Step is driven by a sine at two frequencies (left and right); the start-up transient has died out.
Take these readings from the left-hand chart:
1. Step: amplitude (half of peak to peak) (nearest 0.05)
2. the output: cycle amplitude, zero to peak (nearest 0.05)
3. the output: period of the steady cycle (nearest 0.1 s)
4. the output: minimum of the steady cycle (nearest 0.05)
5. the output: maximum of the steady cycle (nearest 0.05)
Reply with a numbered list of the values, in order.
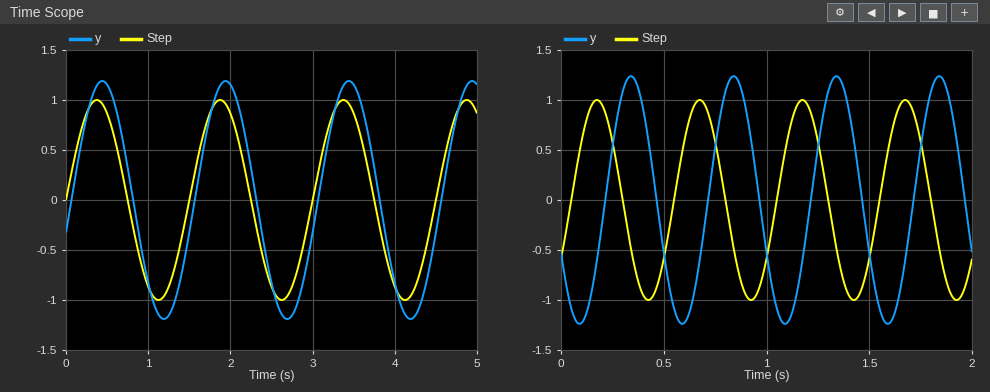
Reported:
1. 1.00
2. 1.20
3. 1.5 s
4. -1.20
5. 1.20
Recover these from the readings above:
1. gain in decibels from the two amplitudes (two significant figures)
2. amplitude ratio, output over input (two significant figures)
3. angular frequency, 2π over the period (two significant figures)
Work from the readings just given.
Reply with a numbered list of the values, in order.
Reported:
1. 1.6 dB
2. 1.2
3. 4.2 rad/s
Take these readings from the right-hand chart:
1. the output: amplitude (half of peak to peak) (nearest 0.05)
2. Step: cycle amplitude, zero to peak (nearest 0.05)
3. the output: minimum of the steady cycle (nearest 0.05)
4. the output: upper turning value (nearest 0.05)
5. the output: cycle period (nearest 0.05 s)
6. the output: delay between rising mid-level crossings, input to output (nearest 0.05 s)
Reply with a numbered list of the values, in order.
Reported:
1. 1.25
2. 1.00
3. -1.25
4. 1.25
5. 0.50 s
6. 0.15 s
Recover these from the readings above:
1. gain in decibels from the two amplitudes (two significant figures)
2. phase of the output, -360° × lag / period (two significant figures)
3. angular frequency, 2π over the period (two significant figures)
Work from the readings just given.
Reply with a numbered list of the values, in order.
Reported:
1. 1.9 dB
2. -110°
3. 13 rad/s
